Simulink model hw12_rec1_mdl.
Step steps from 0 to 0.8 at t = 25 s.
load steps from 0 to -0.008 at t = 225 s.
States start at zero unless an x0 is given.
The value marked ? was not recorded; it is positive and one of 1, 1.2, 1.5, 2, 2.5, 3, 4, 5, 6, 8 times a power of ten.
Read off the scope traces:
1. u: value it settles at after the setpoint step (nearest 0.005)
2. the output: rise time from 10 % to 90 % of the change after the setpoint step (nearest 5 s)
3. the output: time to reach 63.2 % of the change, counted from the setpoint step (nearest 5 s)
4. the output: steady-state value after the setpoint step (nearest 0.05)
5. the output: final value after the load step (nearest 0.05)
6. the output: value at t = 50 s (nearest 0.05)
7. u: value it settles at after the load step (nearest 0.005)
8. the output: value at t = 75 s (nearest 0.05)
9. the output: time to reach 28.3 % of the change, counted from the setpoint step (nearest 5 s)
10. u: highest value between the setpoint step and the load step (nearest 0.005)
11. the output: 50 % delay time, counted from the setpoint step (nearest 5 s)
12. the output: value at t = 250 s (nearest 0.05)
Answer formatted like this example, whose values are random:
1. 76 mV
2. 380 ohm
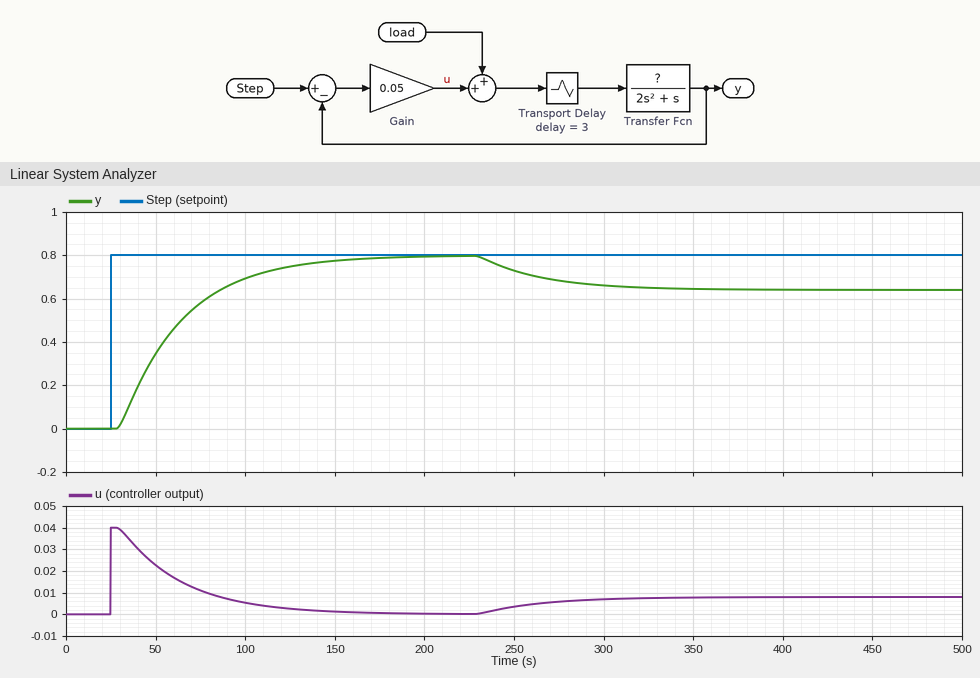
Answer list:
1. 0.000
2. 75 s
3. 40 s
4. 0.80
5. 0.65
6. 0.35
7. 0.010
8. 0.60
9. 15 s
10. 0.040
11. 30 s
12. 0.75
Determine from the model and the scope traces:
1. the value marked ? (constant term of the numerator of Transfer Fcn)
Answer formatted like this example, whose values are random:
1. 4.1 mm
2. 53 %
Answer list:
1. 0.5
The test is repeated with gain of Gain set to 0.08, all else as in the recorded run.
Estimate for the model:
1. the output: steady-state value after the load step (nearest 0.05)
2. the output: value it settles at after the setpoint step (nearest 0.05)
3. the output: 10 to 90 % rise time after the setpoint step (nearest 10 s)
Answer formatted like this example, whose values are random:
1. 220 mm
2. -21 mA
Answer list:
1. 0.70
2. 0.80
3. 40 s
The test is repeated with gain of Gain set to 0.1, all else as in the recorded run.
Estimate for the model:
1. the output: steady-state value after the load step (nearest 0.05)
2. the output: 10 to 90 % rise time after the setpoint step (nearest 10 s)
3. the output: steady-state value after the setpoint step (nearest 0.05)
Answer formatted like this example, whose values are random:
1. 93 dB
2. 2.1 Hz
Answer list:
1. 0.70
2. 30 s
3. 0.80
